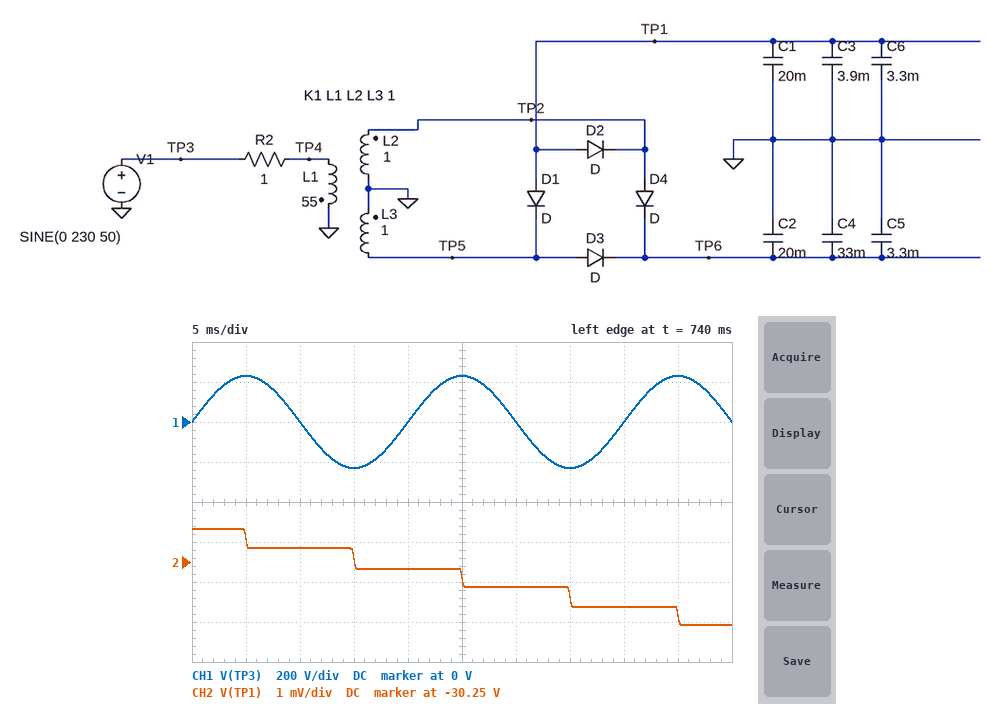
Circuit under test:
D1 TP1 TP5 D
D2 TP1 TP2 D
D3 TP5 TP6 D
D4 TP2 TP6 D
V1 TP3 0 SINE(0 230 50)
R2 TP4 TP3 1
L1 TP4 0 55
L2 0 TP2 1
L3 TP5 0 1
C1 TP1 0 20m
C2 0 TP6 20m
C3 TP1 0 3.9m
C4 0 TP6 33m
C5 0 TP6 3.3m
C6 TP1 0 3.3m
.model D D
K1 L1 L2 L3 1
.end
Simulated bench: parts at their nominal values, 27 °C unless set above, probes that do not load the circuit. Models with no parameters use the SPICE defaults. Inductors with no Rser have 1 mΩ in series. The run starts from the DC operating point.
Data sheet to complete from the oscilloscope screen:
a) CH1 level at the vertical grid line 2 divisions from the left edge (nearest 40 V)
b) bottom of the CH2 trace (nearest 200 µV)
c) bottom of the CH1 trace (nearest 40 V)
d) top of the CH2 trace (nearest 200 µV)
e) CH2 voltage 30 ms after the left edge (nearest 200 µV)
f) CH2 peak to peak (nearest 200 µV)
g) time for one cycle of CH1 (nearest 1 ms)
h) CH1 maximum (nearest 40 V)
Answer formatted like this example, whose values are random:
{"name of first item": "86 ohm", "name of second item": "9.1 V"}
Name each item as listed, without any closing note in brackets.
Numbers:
{"CH1 level at the vertical grid line 2 divisions from the left edge": "0 V", "bottom of the CH2 trace": "-30.2526 V", "bottom of the CH1 trace": "-240 V", "top of the CH2 trace": "-30.2502 V", "CH2 voltage 30 ms after the left edge": "-30.2516 V", "CH2 peak to peak": "2.4 mV", "time for one cycle of CH1": "20 ms", "CH1 maximum": "240 V"}
